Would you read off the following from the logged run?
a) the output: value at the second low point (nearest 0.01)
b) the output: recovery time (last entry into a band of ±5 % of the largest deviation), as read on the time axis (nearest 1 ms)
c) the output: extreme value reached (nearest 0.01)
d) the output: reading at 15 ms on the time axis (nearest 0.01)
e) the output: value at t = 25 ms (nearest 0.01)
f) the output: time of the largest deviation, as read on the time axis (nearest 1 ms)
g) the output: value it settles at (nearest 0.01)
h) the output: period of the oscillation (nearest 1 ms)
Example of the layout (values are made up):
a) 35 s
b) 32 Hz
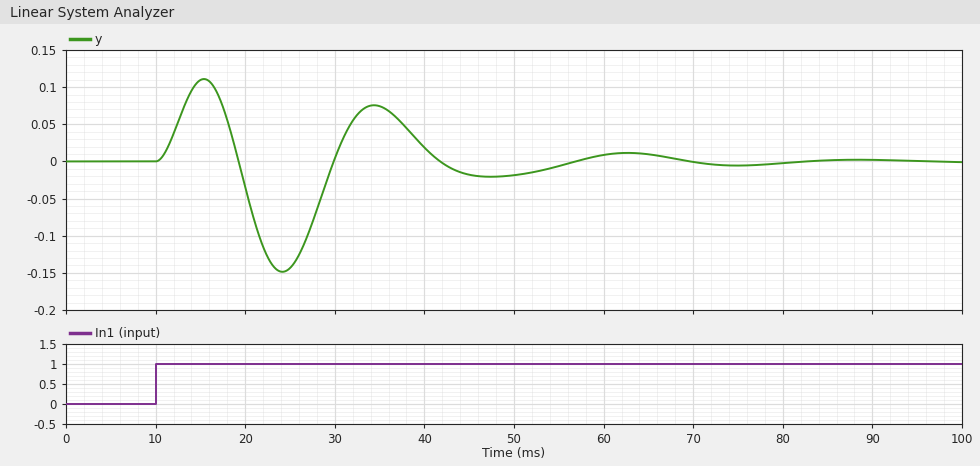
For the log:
a) -0.02
b) 66 ms
c) -0.15
d) 0.11
e) -0.14
f) 24 ms
g) 0.00
h) 23 ms
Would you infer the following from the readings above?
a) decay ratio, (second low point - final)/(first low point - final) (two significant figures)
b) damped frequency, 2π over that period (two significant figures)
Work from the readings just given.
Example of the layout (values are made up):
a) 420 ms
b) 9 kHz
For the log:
a) 0.13
b) 0.27 rad/ms
